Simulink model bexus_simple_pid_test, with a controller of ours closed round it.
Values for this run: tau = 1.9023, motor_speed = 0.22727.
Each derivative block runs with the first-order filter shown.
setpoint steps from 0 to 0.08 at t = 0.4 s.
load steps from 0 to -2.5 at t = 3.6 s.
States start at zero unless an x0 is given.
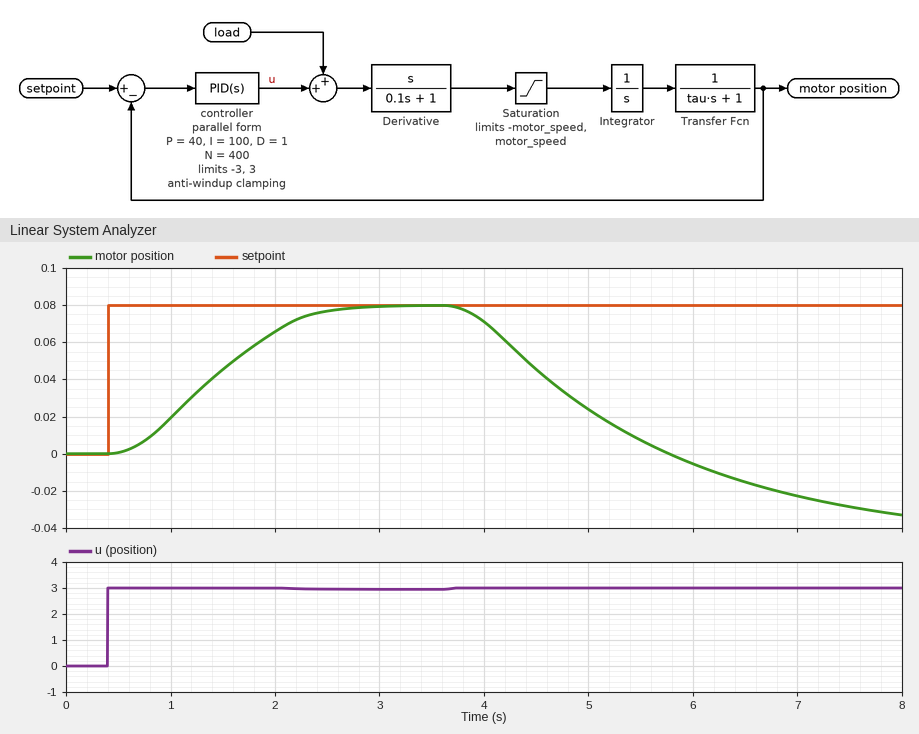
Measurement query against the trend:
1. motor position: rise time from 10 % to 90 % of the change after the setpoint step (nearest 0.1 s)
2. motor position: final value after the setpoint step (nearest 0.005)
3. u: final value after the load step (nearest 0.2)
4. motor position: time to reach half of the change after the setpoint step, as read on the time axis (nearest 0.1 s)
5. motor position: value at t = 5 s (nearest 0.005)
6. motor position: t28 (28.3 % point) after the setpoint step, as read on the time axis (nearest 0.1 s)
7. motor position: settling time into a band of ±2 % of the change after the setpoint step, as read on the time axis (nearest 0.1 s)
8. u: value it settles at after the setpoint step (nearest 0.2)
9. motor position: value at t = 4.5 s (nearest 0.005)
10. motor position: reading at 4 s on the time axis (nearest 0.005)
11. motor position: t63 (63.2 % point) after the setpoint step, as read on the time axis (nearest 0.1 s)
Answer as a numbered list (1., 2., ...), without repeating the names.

1. 1.4 s
2. 0.080
3. 3.0
4. 1.4 s
5. 0.025
6. 1.1 s
7. 2.7 s
8. 3.0
9. 0.045
10. 0.070
11. 1.6 s
